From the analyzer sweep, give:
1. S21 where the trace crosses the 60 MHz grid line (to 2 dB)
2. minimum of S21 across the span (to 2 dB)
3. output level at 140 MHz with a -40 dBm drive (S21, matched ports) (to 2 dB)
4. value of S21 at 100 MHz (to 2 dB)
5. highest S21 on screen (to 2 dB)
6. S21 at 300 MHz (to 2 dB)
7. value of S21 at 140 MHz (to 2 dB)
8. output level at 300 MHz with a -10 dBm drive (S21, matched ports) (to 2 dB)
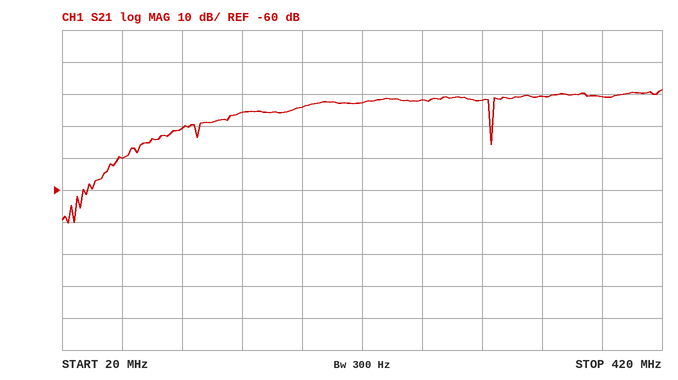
-50 dB
-70 dB
-76 dBm
-40 dB
-28 dB
-32 dB
-36 dB
-42 dBm
